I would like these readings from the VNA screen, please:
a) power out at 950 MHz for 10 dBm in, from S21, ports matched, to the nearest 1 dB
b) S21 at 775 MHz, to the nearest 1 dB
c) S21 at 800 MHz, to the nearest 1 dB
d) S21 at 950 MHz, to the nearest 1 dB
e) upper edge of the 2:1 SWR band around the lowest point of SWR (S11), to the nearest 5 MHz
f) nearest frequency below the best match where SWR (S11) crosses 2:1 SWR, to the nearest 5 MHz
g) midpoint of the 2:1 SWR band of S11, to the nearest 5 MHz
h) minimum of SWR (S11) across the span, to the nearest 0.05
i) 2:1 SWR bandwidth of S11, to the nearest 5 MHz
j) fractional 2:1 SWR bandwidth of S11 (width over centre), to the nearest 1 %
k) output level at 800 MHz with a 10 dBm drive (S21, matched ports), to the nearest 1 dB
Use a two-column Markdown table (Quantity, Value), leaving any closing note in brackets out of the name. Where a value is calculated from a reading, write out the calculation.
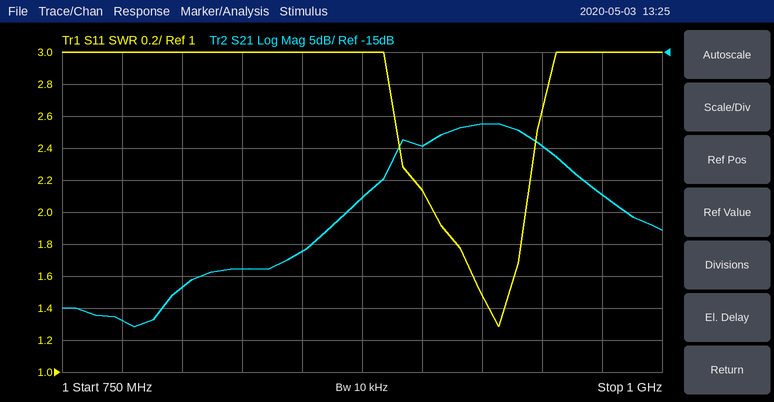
| Quantity | Value |
|---|---|
| power out at 950 MHz for 10 dBm in, from S21, ports matched, to the nearest 1 dB | 10 dBm + (-30 dB) = -20 dBm |
| S21 at 775 MHz, to the nearest 1 dB | -57 dB |
| S21 at 800 MHz, to the nearest 1 dB | -52 dB |
| S21 at 950 MHz, to the nearest 1 dB | -30 dB |
| upper edge of the 2:1 SWR band around the lowest point of SWR (S11), to the nearest 5 MHz | 945 MHz |
| nearest frequency below the best match where SWR (S11) crosses 2:1 SWR, to the nearest 5 MHz | 905 MHz |
| midpoint of the 2:1 SWR band of S11, to the nearest 5 MHz | 925 MHz |
| minimum of SWR (S11) across the span, to the nearest 0.05 | 1.30 |
| 2:1 SWR bandwidth of S11, to the nearest 5 MHz | 945 MHz − 905 MHz = 40 MHz |
| fractional 2:1 SWR bandwidth of S11 (width over centre), to the nearest 1 % | 40 MHz / 925 MHz ≈ 4 % |
| output level at 800 MHz with a 10 dBm drive (S21, matched ports), to the nearest 1 dB | 10 dBm + (-52 dB) = -42 dBm |
